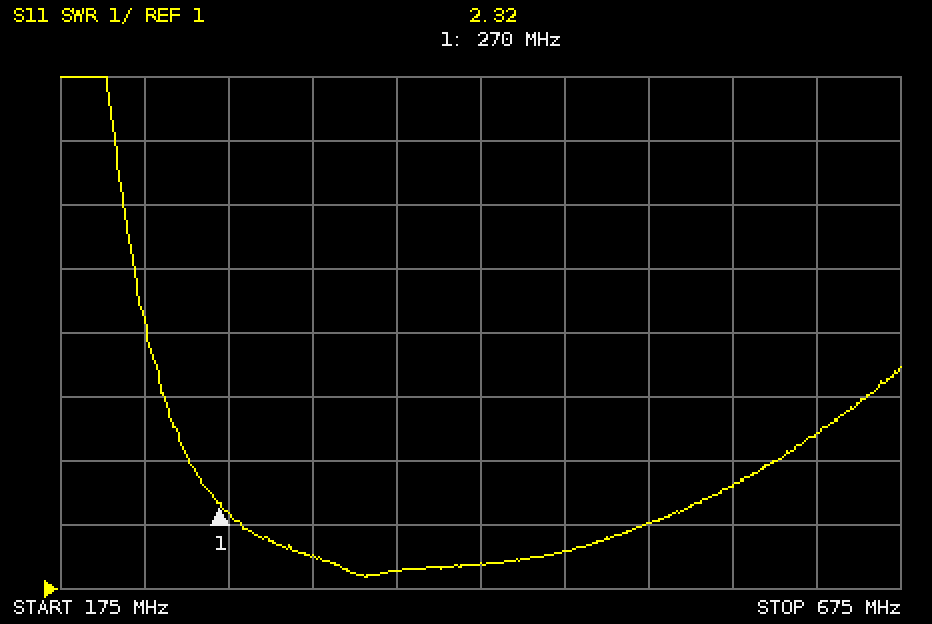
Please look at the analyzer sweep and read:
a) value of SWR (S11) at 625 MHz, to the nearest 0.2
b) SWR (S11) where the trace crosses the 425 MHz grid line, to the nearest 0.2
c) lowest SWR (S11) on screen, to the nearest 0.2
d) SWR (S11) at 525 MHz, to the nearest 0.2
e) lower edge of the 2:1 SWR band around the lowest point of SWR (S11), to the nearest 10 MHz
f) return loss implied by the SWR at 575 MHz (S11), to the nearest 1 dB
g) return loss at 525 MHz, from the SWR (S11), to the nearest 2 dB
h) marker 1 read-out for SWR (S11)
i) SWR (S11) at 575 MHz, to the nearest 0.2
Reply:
3.4
1.4
1.2
2.0
280 MHz
7 dB
10 dB
2.32
2.6
